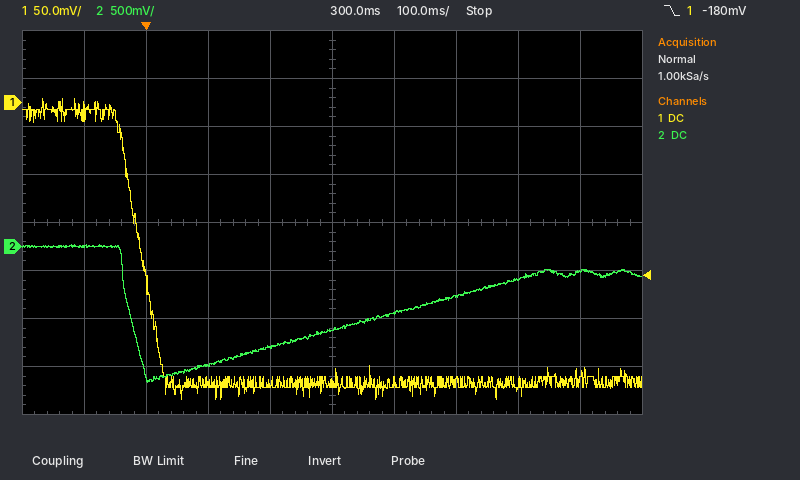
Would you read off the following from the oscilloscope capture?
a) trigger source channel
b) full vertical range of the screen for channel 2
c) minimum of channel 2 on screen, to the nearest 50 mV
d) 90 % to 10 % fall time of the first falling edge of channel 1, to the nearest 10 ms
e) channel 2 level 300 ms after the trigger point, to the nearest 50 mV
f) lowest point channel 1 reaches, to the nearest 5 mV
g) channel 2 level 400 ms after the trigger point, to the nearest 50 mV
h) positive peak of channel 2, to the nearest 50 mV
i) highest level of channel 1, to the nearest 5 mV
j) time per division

channel 1
4 V
-1.40 V
60 ms
-850 mV
-310 mV
-700 mV
0 mV
5 mV
100 ms
